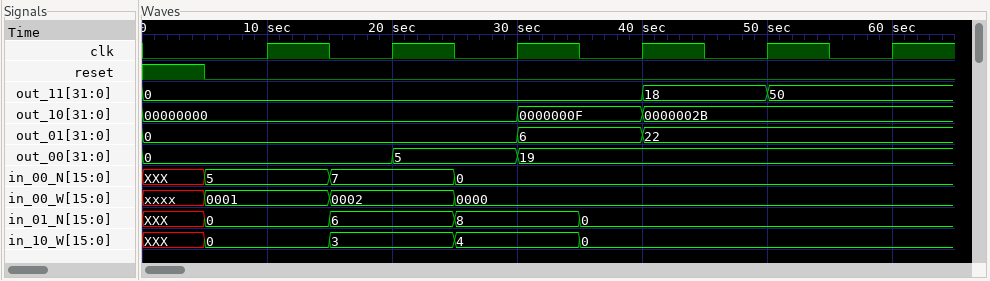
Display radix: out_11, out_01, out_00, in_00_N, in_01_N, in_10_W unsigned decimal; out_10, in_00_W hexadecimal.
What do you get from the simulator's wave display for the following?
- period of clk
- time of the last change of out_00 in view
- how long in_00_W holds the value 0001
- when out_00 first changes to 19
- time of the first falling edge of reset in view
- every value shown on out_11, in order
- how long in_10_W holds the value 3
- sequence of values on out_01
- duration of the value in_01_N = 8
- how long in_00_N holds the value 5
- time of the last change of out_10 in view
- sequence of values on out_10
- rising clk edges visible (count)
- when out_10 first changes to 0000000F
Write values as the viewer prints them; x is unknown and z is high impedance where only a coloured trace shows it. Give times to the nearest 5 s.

10 s
30 s
10 s
30 s
5 s
0, 18, 50
10 s
0, 6, 22
10 s
10 s
40 s
00000000, 0000000F, 0000002B
6
30 s
